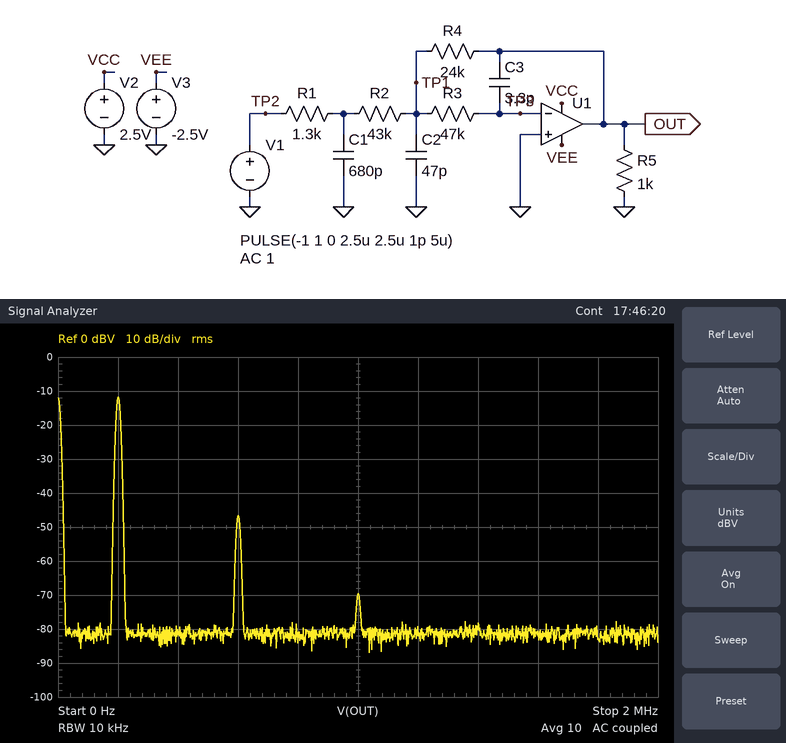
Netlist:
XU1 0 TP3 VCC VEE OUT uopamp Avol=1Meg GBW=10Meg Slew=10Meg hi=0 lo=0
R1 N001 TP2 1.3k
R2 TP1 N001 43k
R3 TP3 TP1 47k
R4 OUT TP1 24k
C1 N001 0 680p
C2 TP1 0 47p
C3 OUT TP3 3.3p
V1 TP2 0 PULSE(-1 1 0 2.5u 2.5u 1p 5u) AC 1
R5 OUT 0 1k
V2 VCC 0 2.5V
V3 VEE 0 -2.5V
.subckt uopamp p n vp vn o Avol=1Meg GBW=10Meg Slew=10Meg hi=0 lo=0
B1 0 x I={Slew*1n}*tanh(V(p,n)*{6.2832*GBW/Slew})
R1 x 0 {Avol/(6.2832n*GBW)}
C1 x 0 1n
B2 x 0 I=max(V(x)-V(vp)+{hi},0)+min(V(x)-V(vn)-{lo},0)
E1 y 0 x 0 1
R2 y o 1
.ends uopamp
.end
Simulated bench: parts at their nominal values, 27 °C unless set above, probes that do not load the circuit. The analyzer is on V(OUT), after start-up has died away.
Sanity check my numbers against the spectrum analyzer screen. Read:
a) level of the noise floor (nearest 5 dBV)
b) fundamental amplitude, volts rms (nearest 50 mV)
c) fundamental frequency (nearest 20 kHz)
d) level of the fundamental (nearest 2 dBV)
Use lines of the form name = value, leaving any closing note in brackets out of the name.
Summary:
level of the noise floor = -80 dBV
fundamental amplitude, volts rms = 250 mV
fundamental frequency = 200 kHz
level of the fundamental = -12 dBV
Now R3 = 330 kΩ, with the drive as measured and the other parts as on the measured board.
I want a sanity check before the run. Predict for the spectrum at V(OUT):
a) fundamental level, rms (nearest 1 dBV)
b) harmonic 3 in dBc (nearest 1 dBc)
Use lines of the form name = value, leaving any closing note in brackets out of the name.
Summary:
fundamental level, rms = -21 dBV
harmonic 3 in dBc = -44 dBc
